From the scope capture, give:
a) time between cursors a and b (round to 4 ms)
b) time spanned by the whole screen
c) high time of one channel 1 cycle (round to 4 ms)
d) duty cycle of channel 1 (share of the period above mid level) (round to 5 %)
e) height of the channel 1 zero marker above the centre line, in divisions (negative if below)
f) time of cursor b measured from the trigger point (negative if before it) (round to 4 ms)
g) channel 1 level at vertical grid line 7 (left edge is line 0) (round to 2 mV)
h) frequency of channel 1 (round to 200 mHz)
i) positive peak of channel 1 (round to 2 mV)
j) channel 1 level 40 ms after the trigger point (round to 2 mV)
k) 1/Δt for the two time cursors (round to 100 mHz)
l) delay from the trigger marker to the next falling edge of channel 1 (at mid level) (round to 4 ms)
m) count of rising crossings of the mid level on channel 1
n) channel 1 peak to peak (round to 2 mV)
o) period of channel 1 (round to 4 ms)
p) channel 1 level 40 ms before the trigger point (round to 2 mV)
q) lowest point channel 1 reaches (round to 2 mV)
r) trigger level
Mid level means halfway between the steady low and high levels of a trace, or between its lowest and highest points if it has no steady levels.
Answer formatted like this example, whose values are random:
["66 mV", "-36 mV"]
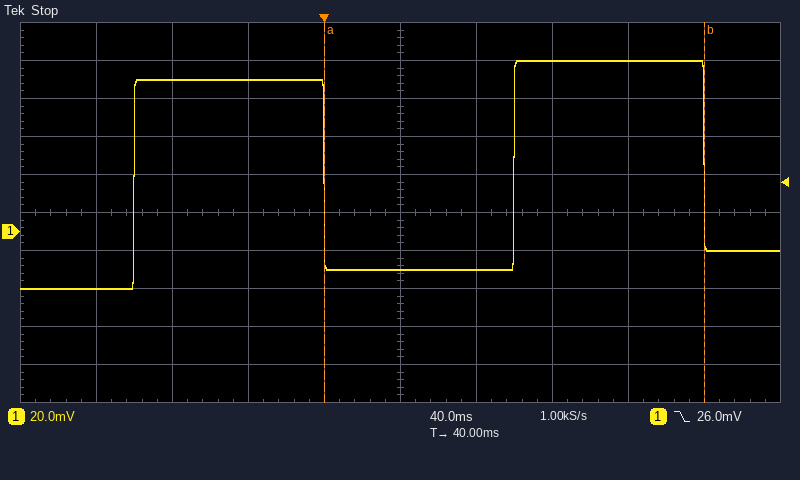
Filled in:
["200 ms", "400 ms", "100 ms", "50 %", "-0.5 div", "+200 ms", "90 mV", "5.0 Hz", "90 mV", "-20 mV", "5.0 Hz", "200 ms", "2", "120 mV", "200 ms", "80 mV", "-30 mV", "26.0 mV"]
